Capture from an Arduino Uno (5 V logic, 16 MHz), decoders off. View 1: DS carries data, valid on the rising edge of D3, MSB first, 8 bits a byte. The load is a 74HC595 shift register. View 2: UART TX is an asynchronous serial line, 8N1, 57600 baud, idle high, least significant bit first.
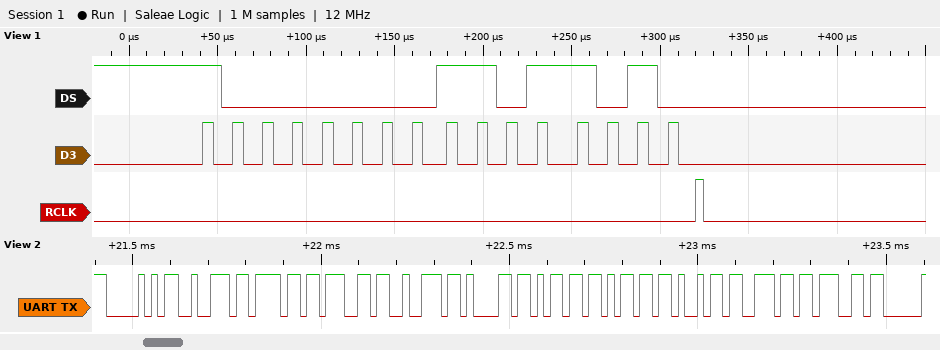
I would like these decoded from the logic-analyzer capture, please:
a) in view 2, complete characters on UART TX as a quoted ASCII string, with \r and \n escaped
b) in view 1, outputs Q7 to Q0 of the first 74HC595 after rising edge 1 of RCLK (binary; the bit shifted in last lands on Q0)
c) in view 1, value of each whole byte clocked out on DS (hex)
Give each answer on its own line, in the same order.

"Programming"
11011010
0x80 0xDA
